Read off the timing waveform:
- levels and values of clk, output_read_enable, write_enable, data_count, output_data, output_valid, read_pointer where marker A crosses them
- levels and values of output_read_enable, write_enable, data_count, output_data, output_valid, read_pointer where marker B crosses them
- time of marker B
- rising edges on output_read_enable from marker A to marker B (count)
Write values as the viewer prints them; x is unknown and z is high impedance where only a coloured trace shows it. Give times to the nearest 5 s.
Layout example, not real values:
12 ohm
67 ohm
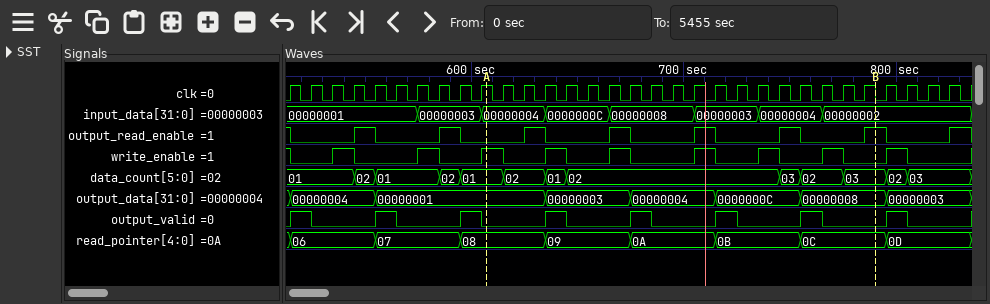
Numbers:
clk=1, output_read_enable=0, write_enable=1, data_count=01, output_data=00000001, output_valid=0, read_pointer=08
output_read_enable=1, write_enable=0, data_count=03, output_data=00000008, output_valid=0, read_pointer=0C
790 s
5
